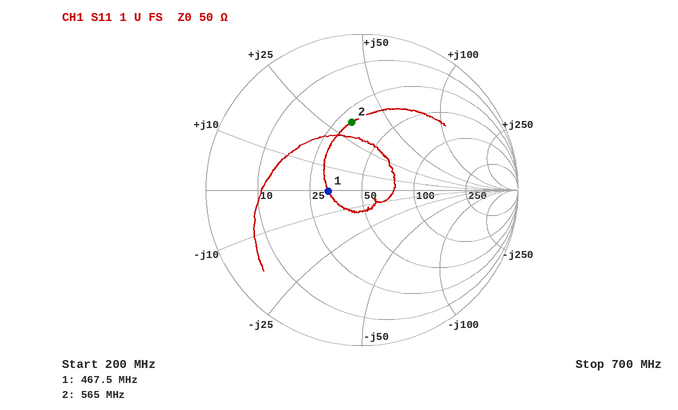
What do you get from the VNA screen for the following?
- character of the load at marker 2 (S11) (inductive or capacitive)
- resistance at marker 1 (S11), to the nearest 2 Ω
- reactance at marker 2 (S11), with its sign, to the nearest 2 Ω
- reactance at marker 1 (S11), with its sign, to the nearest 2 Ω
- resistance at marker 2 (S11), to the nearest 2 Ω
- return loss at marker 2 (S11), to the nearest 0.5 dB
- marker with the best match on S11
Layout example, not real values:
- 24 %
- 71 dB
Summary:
- inductive
- 32 Ω
- +32 Ω
- 0 Ω
- 30 Ω
- 7.0 dB
- marker 1
